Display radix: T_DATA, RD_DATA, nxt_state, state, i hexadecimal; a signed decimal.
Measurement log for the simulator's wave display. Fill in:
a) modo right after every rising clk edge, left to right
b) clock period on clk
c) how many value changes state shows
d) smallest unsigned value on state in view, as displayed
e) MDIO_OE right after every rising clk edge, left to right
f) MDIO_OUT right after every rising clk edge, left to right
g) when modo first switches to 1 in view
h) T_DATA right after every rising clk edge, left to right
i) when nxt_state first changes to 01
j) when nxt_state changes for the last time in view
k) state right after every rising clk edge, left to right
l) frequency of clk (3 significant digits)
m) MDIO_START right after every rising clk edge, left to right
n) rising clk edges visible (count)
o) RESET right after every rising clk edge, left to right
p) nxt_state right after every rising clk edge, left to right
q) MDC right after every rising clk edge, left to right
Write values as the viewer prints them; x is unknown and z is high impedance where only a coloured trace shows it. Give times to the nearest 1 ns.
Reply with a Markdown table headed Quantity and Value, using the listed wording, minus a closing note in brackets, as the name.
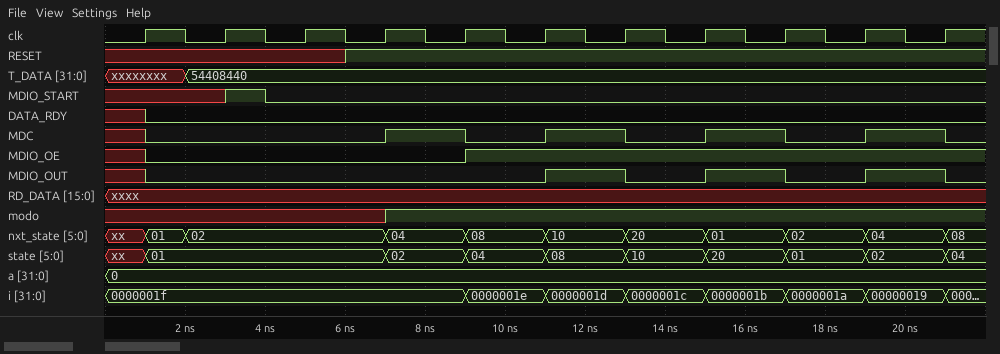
| Quantity | Value |
|---|---|
| modo right after every rising clk edge, left to right | x x x 1 1 1 1 1 1 1 1 |
| clock period on clk | 2 ns |
| how many value changes state shows | 9 |
| smallest unsigned value on state in view, as displayed | 01 |
| MDIO_OE right after every rising clk edge, left to right | 0 0 0 0 1 1 1 1 1 1 1 |
| MDIO_OUT right after every rising clk edge, left to right | 0 0 0 0 0 1 0 1 0 1 0 |
| when modo first switches to 1 in view | 7 ns |
| T_DATA right after every rising clk edge, left to right | xxxxxxxx, 54408440, 54408440, 54408440, 54408440, 54408440, 54408440, 54408440, 54408440, 54408440, 54408440 |
| when nxt_state first changes to 01 | 1 ns |
| when nxt_state changes for the last time in view | 21 ns |
| state right after every rising clk edge, left to right | 01, 01, 01, 02, 04, 08, 10, 20, 01, 02, 04 |
| frequency of clk | 500 MHz |
| MDIO_START right after every rising clk edge, left to right | x 1 0 0 0 0 0 0 0 0 0 |
| rising clk edges visible | 11 |
| RESET right after every rising clk edge, left to right | x x x 1 1 1 1 1 1 1 1 |
| nxt_state right after every rising clk edge, left to right | 01, 02, 02, 04, 08, 10, 20, 01, 02, 04, 08 |
| MDC right after every rising clk edge, left to right | 0 0 0 1 0 1 0 1 0 1 0 |
